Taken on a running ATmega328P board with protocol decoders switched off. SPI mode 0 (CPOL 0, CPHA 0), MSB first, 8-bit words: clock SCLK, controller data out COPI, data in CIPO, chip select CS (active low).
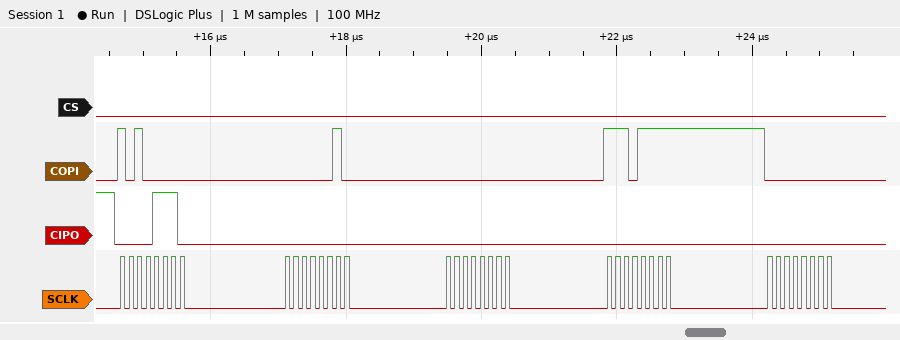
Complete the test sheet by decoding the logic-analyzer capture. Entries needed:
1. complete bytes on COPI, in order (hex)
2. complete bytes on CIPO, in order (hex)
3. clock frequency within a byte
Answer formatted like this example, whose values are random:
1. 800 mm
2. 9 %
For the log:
1. A0 02 00 EF 00
2. 0E 00 00 00 00
3. 8 MHz
